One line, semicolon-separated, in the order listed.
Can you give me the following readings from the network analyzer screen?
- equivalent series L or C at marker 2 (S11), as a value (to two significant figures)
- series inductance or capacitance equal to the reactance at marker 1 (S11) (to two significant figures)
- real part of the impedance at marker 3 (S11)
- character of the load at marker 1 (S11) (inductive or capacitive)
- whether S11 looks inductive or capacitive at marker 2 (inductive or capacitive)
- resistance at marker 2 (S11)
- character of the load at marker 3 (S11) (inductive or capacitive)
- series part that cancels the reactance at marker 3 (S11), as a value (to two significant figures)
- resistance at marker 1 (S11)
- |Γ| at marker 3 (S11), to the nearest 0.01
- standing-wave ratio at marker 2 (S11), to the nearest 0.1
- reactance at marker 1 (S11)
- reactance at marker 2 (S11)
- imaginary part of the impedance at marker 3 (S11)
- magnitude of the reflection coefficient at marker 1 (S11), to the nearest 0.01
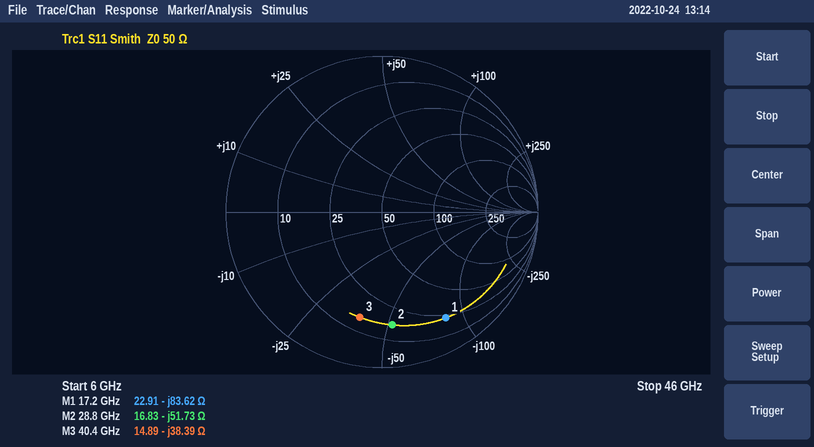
110 fF; 110 fF; 14.89 Ω; capacitive; capacitive; 16.83 Ω; capacitive; 150 pH; 22.91 Ω; 0.69; 6.3; -83.62 Ω; -51.73 Ω; -38.39 Ω; 0.79
